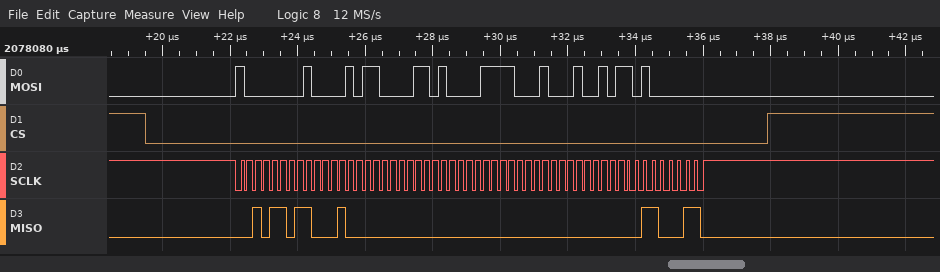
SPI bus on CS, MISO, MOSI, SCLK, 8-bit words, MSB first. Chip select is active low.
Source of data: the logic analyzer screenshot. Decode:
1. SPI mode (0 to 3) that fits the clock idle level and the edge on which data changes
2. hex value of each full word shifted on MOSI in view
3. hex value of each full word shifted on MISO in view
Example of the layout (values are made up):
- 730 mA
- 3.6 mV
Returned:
- 3
- 80, 85, 86, 87, 88, 96, 80
- 2D, 88, 00, 00, 00, 00, C6
